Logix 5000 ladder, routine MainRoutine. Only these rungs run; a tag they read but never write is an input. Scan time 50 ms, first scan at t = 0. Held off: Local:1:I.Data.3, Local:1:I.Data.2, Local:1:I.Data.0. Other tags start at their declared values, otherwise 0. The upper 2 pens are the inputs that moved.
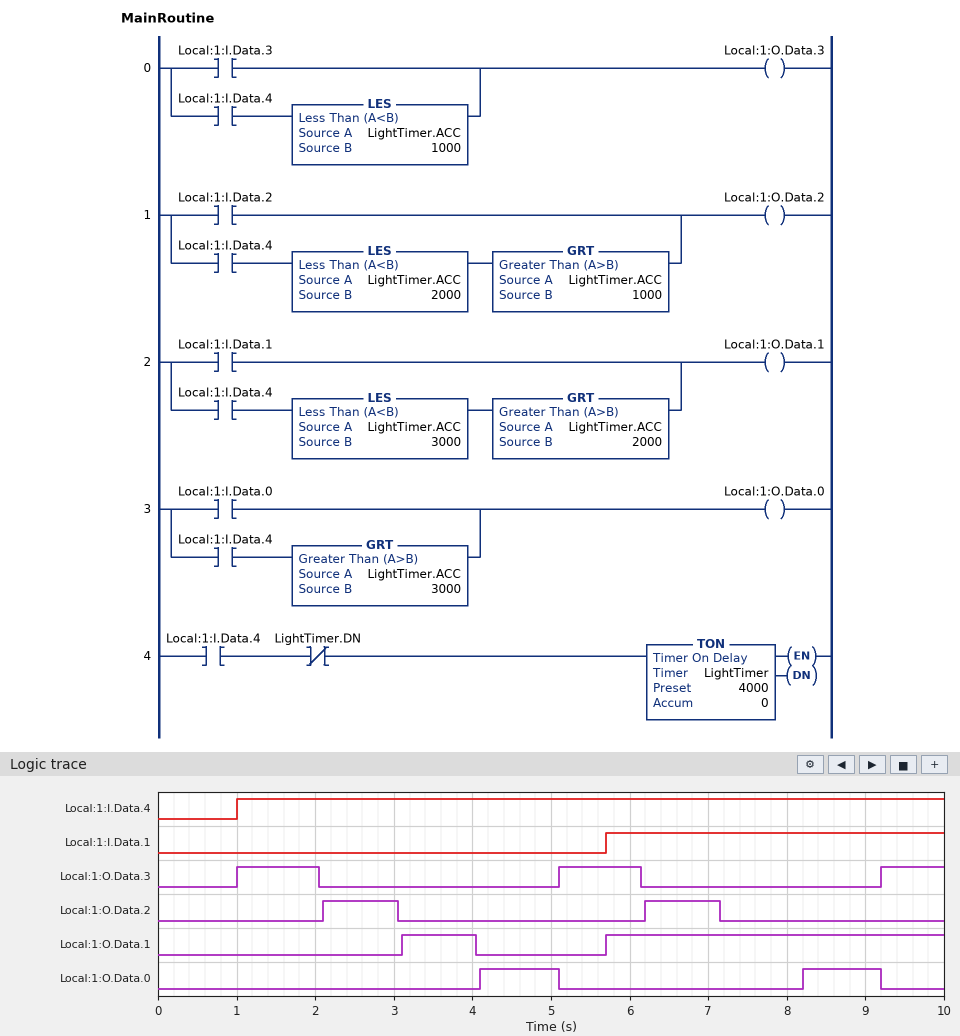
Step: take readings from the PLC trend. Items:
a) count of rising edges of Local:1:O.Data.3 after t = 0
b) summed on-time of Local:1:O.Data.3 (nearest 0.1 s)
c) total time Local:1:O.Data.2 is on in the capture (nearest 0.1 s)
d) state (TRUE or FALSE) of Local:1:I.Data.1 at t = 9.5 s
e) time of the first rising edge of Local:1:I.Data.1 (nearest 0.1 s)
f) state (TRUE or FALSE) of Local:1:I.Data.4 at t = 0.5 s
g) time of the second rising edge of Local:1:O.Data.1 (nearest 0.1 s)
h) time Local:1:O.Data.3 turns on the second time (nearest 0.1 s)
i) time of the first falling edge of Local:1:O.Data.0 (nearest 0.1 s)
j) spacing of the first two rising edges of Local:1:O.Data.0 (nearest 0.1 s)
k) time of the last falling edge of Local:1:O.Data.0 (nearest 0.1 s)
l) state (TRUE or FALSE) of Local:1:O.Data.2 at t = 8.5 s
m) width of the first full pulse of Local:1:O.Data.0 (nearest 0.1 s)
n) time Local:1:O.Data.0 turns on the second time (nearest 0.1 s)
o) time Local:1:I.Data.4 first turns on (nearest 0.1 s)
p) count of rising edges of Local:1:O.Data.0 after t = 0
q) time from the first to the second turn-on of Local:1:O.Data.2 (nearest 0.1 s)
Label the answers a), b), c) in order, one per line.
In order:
a) 3
b) 2.9 s
c) 1.9 s
d) TRUE
e) 5.7 s
f) FALSE
g) 5.7 s
h) 5.1 s
i) 5.1 s
j) 4.1 s
k) 9.2 s
l) FALSE
m) 1.0 s
n) 8.2 s
o) 1.0 s
p) 2
q) 4.1 s
